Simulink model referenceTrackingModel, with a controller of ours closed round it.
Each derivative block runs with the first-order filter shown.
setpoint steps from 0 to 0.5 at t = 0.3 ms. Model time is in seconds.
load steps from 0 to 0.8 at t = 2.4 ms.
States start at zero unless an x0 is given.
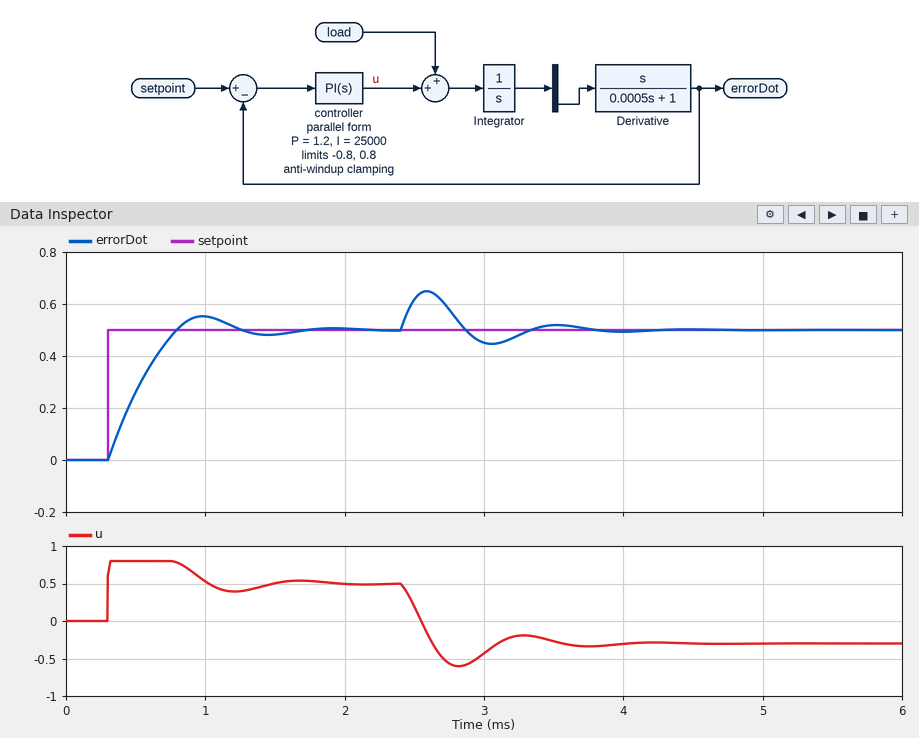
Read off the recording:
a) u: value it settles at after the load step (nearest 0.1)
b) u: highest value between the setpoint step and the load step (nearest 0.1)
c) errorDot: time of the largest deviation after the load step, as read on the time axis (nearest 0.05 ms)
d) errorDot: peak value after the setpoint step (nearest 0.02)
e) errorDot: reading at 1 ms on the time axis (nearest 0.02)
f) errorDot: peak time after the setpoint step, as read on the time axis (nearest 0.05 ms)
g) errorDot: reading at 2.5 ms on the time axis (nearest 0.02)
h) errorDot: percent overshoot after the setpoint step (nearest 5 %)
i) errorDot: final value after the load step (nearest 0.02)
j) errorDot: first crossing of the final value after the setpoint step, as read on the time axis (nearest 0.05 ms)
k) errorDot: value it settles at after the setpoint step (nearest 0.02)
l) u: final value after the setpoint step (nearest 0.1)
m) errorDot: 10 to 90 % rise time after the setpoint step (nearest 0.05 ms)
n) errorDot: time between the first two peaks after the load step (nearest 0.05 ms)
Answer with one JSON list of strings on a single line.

["-0.3", "0.8", "2.60 ms", "0.56", "0.56", "1.00 ms", "0.62", "10 %", "0.50", "0.80 ms", "0.50", "0.5", "0.40 ms", "0.95 ms"]
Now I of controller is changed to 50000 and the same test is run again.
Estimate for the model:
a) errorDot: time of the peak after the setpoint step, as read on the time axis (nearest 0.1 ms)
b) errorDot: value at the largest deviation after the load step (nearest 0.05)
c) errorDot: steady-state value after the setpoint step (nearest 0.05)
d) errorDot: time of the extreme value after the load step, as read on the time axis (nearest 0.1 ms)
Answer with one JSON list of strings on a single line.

["0.9 ms", "0.60", "0.50", "2.5 ms"]
